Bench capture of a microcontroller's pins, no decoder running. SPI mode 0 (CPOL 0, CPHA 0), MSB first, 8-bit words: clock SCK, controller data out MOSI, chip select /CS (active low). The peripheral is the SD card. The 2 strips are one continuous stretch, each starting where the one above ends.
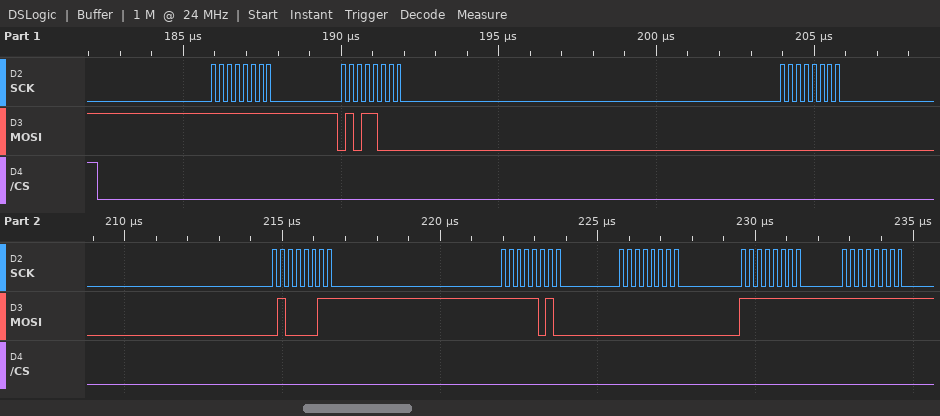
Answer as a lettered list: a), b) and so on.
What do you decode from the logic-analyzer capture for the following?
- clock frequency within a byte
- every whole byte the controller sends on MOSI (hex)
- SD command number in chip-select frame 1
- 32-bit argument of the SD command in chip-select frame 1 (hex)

a) 4 MHz
b) FF 58 00 43 FA 00 FF FF
c) CMD24
d) 0x0043FA00
